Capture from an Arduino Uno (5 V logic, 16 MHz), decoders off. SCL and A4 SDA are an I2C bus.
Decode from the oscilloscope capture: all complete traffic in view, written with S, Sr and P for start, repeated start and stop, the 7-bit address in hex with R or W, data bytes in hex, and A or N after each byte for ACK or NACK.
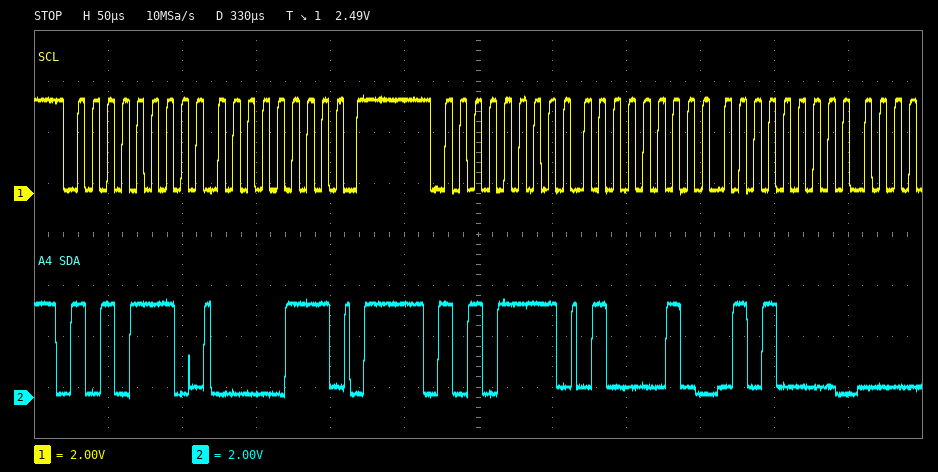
S 57W A 07 A P S 57R A 42 A 50 A
